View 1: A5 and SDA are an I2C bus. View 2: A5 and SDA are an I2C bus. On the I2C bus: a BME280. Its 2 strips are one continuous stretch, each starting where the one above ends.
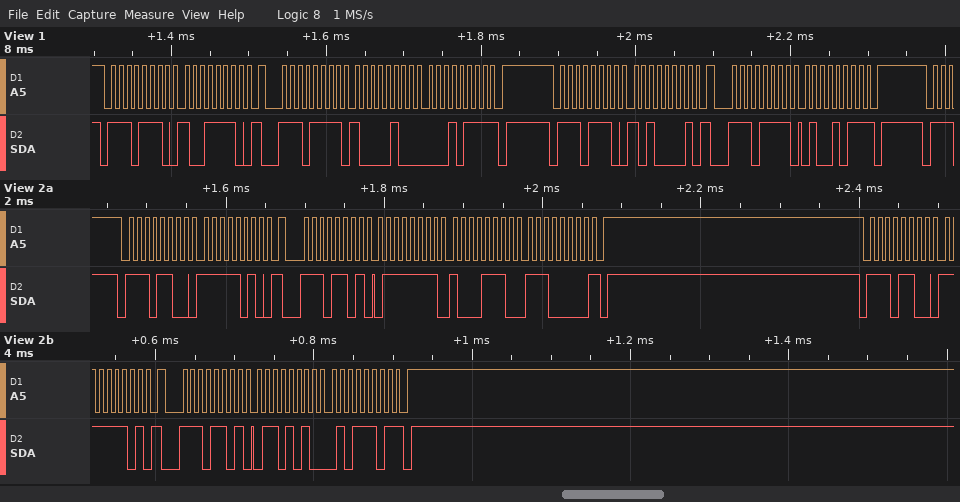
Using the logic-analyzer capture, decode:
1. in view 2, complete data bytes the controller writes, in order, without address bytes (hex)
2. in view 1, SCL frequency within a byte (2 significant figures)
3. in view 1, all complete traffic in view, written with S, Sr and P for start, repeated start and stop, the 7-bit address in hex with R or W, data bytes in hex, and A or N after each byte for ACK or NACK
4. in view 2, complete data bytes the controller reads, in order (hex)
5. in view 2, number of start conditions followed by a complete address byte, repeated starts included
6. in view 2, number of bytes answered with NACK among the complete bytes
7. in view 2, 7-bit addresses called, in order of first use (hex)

FA FD
100 kHz
S 77W A 9E A Sr 77R A 84 A 17 N P S 77W A A1 A Sr 77R A 4B N P
7F 8E E0 6A 5D
4
2
0x76
